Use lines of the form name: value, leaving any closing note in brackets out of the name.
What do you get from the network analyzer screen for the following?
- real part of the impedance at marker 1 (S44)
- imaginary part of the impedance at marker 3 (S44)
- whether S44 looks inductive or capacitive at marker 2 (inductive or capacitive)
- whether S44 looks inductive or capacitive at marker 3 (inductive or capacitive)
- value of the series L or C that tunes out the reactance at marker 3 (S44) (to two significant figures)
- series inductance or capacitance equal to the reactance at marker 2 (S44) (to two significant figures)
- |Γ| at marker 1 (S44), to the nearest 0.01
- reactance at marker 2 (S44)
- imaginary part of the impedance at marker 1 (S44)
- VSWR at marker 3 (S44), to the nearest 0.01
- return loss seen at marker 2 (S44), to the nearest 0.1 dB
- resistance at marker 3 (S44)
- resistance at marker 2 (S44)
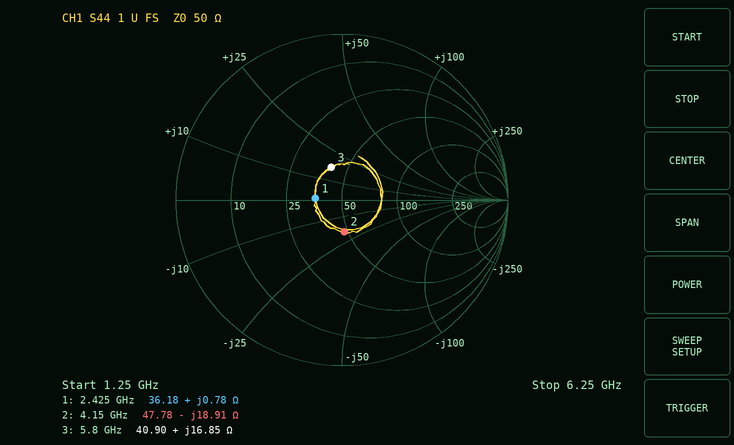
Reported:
real part of the impedance at marker 1: 36.18 Ω
imaginary part of the impedance at marker 3: +16.85 Ω
whether S44 looks inductive or capacitive at marker 2: capacitive
whether S44 looks inductive or capacitive at marker 3: inductive
value of the series L or C that tunes out the reactance at marker 3 (S44): 1.6 pF
series inductance or capacitance equal to the reactance at marker 2 (S44): 2.0 pF
|Γ| at marker 1 (S44), to the nearest 0.01: 0.16
reactance at marker 2: -18.91 Ω
imaginary part of the impedance at marker 1: +0.78 Ω
VSWR at marker 3 (S44), to the nearest 0.01: 1.52
return loss seen at marker 2 (S44), to the nearest 0.1 dB: 14.4 dB
resistance at marker 3: 40.90 Ω
resistance at marker 2: 47.78 Ω
